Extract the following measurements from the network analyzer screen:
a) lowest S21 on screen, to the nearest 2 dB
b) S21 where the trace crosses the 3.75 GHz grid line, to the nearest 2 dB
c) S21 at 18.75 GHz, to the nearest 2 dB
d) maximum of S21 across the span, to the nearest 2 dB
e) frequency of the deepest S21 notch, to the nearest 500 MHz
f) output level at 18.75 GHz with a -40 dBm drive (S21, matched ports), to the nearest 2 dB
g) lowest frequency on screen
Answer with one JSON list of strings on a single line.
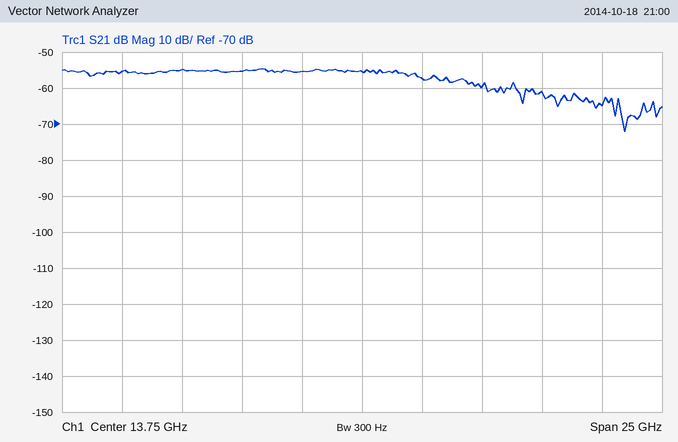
["-72 dB", "-56 dB", "-60 dB", "-54 dB", "24.5 GHz", "-100 dBm", "1.25 GHz"]
